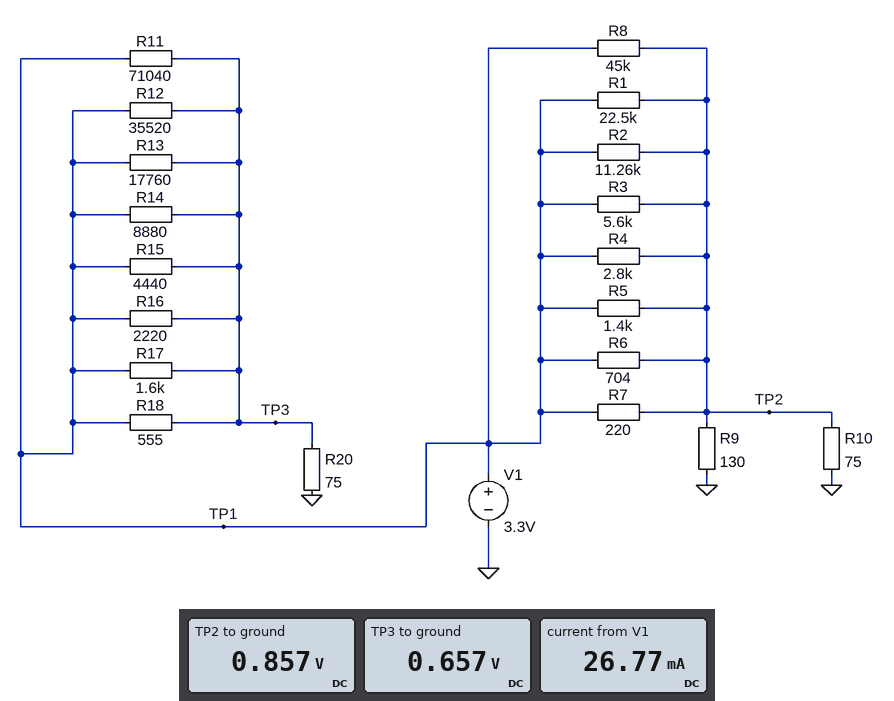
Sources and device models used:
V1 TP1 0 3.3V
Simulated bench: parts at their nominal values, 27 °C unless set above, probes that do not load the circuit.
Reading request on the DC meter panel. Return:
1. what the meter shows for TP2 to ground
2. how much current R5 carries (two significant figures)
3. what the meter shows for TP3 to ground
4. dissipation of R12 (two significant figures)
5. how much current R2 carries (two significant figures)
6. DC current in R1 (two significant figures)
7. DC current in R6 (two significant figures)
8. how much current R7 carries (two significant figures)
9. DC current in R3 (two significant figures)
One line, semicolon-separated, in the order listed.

0.857 V; 1.7 mA; 0.657 V; 200 µW; 220 µA; 110 µA; 3.5 mA; 11 mA; 440 µA
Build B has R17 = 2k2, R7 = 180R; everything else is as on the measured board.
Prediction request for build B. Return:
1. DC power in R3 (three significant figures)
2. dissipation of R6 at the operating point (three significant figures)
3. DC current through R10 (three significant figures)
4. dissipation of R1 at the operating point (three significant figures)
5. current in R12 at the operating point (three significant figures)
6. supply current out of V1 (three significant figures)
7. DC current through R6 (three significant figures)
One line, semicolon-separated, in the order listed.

994 µW; 7.91 mW; 12.5 mA; 247 µW; 75.2 µA; 28.2 mA; 3.35 mA
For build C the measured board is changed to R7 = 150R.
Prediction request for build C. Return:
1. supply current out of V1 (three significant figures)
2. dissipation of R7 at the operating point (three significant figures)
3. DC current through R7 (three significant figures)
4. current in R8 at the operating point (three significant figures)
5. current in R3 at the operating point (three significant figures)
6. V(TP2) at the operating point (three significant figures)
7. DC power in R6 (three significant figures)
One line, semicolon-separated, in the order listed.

30.3 mA; 34.5 mW; 15.2 mA; 50.5 µA; 406 µA; 1.03 V; 7.34 mW
